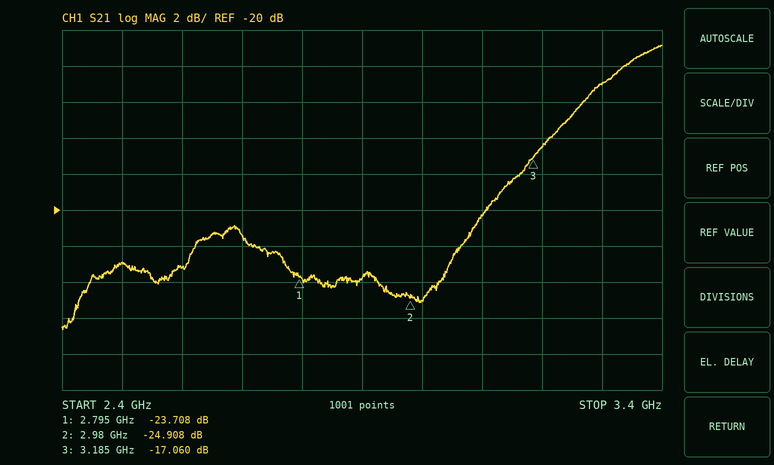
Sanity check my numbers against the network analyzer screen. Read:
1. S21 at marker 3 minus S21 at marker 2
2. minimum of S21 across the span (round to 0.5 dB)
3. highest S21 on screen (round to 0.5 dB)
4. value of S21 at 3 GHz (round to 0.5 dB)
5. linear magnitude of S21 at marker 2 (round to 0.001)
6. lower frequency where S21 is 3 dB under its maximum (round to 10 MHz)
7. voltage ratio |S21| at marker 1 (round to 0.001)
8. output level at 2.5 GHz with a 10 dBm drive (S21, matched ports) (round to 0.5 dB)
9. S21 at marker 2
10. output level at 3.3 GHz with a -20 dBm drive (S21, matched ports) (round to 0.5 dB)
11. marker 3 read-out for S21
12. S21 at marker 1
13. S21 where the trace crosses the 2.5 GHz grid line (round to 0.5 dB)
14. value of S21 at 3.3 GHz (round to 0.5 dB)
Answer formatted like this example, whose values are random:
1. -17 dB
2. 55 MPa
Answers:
1. 7.848 dB
2. -26.5 dB
3. -11.0 dB
4. -25.0 dB
5. 0.057
6. 3.27 GHz
7. 0.065
8. -13.0 dBm
9. -24.908 dB
10. -33.0 dBm
11. -17.060 dB
12. -23.708 dB
13. -23.0 dB
14. -13.0 dB
